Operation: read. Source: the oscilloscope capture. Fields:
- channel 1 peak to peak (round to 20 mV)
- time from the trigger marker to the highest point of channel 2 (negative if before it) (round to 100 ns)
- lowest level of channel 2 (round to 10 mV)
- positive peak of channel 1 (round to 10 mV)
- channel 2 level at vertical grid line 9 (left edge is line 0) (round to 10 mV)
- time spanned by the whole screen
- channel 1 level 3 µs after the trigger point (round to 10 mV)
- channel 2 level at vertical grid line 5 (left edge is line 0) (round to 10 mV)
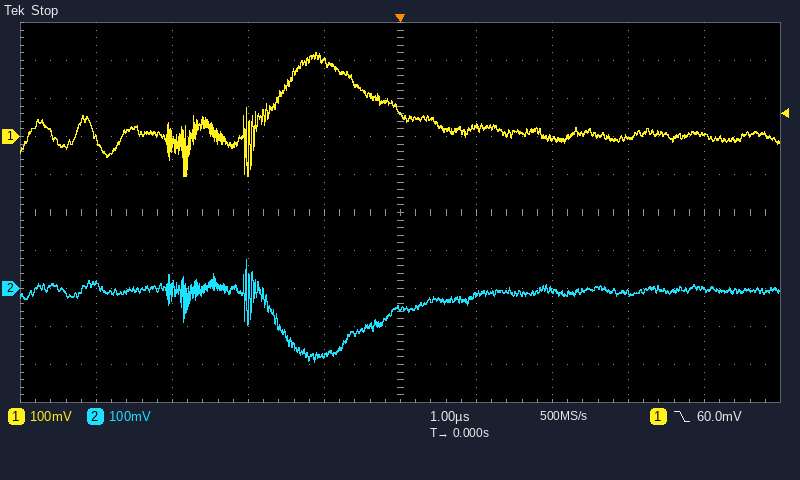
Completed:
320 mV
-2.0 µs
-190 mV
220 mV
0 mV
10 µs
0 mV
-50 mV
